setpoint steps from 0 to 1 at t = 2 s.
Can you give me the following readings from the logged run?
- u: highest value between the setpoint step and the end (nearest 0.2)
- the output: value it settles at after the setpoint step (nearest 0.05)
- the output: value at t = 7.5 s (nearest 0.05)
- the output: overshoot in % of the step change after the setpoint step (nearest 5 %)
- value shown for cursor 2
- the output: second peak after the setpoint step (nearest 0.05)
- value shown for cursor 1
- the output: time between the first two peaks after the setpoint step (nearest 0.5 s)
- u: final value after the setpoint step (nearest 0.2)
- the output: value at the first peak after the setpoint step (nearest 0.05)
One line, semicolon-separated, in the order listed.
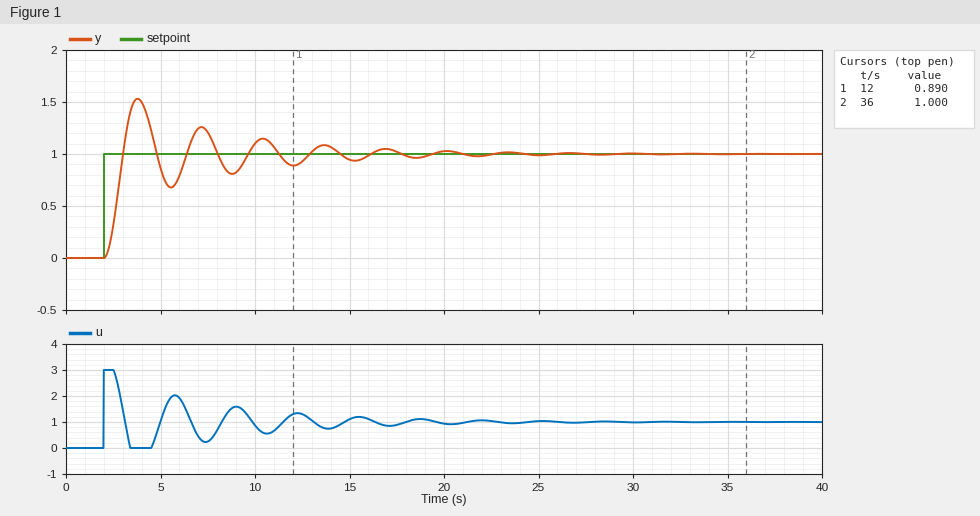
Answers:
3.0; 1.00; 1.20; 55 %; 1.000; 1.25; 0.890; 3.5 s; 1.0; 1.55
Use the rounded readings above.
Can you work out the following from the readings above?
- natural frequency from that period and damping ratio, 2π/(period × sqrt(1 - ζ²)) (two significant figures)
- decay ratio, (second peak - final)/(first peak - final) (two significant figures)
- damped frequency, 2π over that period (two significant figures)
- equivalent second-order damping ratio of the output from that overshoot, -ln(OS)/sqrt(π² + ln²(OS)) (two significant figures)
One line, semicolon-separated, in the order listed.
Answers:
1.8 rad/s; 0.45; 1.8 rad/s; 0.19
